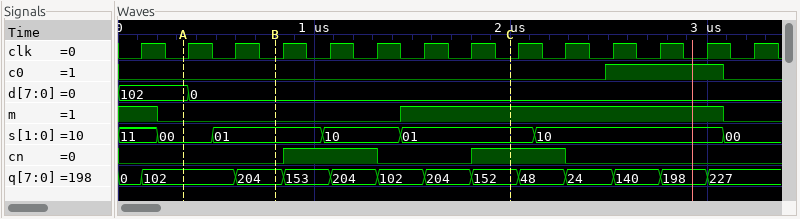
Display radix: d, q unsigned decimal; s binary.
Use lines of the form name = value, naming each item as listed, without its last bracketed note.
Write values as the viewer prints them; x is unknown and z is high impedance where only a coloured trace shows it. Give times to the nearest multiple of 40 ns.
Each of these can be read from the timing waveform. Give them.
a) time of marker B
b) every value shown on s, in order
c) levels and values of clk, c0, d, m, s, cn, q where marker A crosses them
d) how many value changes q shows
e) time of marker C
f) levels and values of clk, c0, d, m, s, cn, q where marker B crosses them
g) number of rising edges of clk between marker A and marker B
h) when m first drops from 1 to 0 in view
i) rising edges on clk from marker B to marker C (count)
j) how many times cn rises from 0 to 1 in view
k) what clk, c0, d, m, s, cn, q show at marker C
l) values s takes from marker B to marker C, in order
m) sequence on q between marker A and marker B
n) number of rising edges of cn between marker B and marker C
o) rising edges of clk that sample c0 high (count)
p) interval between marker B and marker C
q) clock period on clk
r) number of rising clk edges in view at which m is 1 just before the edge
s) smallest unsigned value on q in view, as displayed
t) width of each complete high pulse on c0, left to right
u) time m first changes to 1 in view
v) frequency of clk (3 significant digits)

time of marker B = 800 ns
every value shown on s, in order = 11, 00, 01, 10, 01, 10, 00
levels and values of clk, c0, d, m, s, cn, q where marker A crosses them = clk=0, c0=0, d=102, m=0, s=00, cn=0, q=102
how many value changes q shows = 12
time of marker C = 2000 ns
levels and values of clk, c0, d, m, s, cn, q where marker B crosses them = clk=0, c0=0, d=0, m=0, s=01, cn=0, q=204
number of rising edges of clk between marker A and marker B = 2
when m first drops from 1 to 0 in view = 200 ns
rising edges on clk from marker B to marker C = 5
how many times cn rises from 0 to 1 in view = 2
what clk, c0, d, m, s, cn, q show at marker C = clk=0, c0=0, d=0, m=1, s=01, cn=1, q=152
values s takes from marker B to marker C, in order = 01, 10, 01
sequence on q between marker A and marker B = 102, 204
number of rising edges of cn between marker B and marker C = 2
rising edges of clk that sample c0 high = 3
interval between marker B and marker C = 1200 ns
clock period on clk = 240 ns
number of rising clk edges in view at which m is 1 just before the edge = 8
smallest unsigned value on q in view, as displayed = 0
width of each complete high pulse on c0, left to right = 600 ns
time m first changes to 1 in view = 1440 ns
frequency of clk = 4.17 MHz
